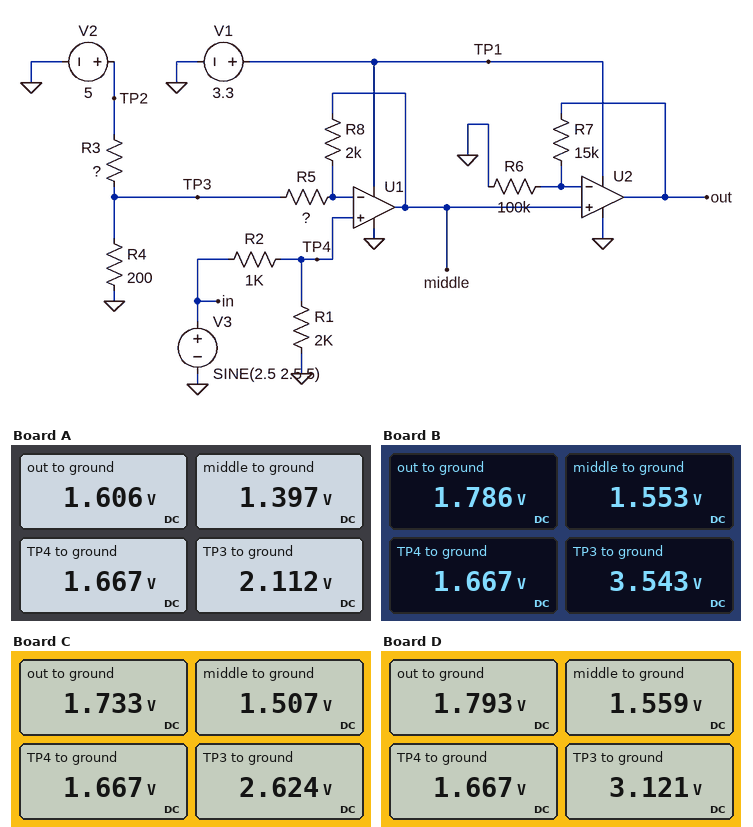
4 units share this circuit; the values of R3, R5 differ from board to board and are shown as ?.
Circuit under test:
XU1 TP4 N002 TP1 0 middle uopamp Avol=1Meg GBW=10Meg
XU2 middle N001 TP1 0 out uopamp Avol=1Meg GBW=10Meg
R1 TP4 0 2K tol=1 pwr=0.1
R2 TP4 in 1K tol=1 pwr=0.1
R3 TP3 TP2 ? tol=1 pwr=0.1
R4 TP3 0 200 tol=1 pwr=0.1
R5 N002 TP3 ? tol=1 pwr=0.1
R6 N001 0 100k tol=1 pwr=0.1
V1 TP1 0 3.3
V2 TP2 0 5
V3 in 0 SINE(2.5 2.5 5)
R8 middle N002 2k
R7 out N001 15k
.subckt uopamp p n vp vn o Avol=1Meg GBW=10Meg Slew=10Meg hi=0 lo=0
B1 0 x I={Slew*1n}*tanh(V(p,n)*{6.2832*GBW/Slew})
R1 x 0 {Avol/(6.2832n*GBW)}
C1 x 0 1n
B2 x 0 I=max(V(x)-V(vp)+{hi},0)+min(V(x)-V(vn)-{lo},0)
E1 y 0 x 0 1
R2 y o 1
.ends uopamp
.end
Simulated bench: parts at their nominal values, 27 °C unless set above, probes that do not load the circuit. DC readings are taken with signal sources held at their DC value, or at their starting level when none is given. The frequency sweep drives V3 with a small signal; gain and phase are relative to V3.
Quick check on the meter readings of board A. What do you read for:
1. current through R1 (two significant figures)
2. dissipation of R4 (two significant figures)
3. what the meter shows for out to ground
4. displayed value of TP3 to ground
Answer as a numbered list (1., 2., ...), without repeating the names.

1. 830 µA
2. 22 mW
3. 1.606 V
4. 2.112 V
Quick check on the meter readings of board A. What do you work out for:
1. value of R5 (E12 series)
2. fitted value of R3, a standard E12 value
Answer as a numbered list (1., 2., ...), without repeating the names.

1. 3.3 kΩ
2. 270 Ω
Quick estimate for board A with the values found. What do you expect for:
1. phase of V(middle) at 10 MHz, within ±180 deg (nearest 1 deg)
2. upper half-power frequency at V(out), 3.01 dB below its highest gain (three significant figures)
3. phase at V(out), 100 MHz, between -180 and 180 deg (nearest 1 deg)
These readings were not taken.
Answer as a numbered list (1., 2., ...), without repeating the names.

1. -58 deg
2. 4.68 MHz
3. -171 deg
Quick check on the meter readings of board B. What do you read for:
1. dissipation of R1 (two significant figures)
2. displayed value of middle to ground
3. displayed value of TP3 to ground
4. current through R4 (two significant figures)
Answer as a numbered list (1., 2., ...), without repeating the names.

1. 1.4 mW
2. 1.553 V
3. 3.543 V
4. 18 mA
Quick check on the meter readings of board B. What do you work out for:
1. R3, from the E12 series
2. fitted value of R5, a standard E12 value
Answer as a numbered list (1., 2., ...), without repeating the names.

1. 82 Ω
2. 33 kΩ
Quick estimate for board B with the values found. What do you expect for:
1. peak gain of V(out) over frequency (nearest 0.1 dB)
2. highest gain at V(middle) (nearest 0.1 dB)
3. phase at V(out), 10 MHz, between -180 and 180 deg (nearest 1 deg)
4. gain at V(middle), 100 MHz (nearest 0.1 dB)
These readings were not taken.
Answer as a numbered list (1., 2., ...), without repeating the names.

1. -1.8 dB
2. -3.0 dB
3. -96 deg
4. -23.6 dB
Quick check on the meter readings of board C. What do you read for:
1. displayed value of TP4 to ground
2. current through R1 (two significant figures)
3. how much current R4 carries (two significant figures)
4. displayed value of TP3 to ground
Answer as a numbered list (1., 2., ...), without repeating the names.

1. 1.667 V
2. 830 µA
3. 13 mA
4. 2.624 V
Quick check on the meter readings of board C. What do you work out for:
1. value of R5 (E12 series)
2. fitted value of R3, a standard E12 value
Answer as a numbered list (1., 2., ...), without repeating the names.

1. 12 kΩ
2. 180 Ω
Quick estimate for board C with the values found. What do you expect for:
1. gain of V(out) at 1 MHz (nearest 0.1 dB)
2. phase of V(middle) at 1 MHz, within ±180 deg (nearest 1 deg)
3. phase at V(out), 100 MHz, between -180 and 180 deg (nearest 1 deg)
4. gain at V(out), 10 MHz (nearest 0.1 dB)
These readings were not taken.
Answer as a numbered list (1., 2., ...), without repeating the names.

1. -1.1 dB
2. -7 deg
3. -170 deg
4. -8.4 dB
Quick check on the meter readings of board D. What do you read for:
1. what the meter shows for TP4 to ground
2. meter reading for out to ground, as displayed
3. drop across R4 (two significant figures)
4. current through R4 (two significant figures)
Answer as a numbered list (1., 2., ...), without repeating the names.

1. 1.667 V
2. 1.793 V
3. 3.1 V
4. 16 mA
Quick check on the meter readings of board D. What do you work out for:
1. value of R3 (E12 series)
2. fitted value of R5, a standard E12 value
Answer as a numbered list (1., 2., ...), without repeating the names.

1. 120 Ω
2. 27 kΩ
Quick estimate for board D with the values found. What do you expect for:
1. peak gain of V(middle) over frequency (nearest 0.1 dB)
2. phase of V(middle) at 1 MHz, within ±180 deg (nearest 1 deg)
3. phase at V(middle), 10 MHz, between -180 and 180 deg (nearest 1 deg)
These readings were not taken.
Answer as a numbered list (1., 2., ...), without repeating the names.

1. -2.9 dB
2. -6 deg
3. -47 deg
